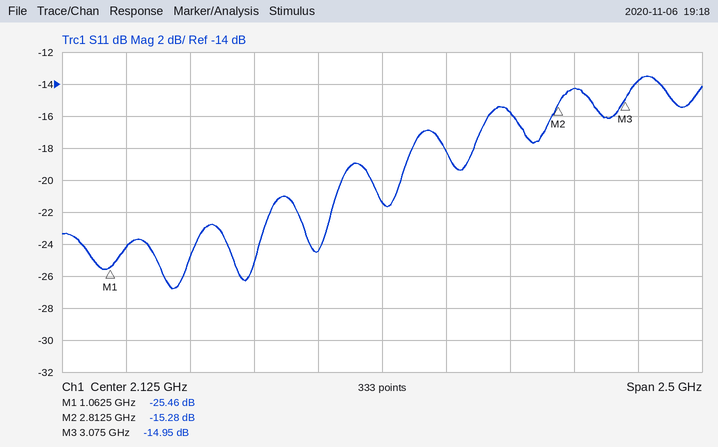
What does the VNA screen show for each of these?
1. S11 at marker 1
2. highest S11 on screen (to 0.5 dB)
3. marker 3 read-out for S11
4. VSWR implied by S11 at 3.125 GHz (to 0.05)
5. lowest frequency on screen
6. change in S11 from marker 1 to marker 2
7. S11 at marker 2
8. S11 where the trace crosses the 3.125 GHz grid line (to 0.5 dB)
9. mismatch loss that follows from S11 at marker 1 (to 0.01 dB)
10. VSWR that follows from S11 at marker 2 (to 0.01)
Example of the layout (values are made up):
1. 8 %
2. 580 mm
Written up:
1. -25.46 dB
2. -13.5 dB
3. -14.95 dB
4. 1.50
5. 875 MHz
6. 10.18 dB
7. -15.28 dB
8. -14.0 dB
9. 0.01 dB
10. 1.42
